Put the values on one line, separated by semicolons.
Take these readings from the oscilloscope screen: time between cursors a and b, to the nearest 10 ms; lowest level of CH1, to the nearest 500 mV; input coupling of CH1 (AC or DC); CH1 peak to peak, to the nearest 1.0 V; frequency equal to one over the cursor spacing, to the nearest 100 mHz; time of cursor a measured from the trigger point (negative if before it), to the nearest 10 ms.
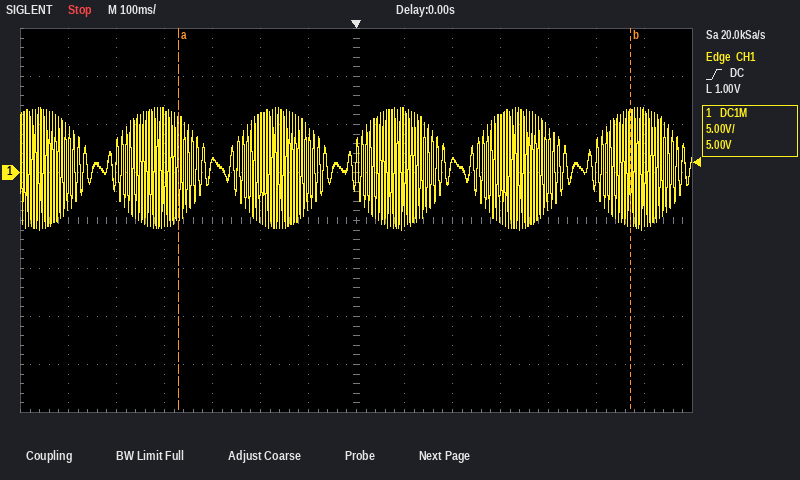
940 ms; -6.0 V; DC; 13.0 V; 1.1 Hz; -370 ms
